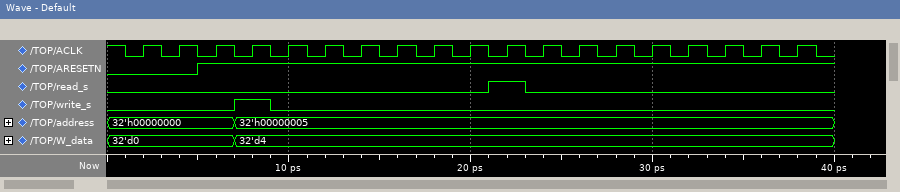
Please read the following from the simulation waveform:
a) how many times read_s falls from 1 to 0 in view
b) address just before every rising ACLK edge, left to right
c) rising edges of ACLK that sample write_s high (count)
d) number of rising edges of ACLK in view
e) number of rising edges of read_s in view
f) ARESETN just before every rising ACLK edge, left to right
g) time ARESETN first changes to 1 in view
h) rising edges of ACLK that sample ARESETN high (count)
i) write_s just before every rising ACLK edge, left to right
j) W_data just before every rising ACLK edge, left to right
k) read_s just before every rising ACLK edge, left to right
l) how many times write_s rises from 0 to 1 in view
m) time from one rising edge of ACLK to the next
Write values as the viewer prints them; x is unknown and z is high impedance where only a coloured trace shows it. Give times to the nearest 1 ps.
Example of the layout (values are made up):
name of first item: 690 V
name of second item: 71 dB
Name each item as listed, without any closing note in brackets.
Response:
how many times read_s falls from 1 to 0 in view: 1
address just before every rising ACLK edge, left to right: 32'h00000000, 32'h00000000, 32'h00000000, 32'h00000005, 32'h00000005, 32'h00000005, 32'h00000005, 32'h00000005, 32'h00000005, 32'h00000005, 32'h00000005, 32'h00000005, 32'h00000005, 32'h00000005, 32'h00000005, 32'h00000005, 32'h00000005, 32'h00000005, 32'h00000005
rising edges of ACLK that sample write_s high: 1
number of rising edges of ACLK in view: 19
number of rising edges of read_s in view: 1
ARESETN just before every rising ACLK edge, left to right: 0 0 1 1 1 1 1 1 1 1 1 1 1 1 1 1 1 1 1
time ARESETN first changes to 1 in view: 5 ps
rising edges of ACLK that sample ARESETN high: 17
write_s just before every rising ACLK edge, left to right: 0 0 0 1 0 0 0 0 0 0 0 0 0 0 0 0 0 0 0
W_data just before every rising ACLK edge, left to right: 32'd0, 32'd0, 32'd0, 32'd4, 32'd4, 32'd4, 32'd4, 32'd4, 32'd4, 32'd4, 32'd4, 32'd4, 32'd4, 32'd4, 32'd4, 32'd4, 32'd4, 32'd4, 32'd4
read_s just before every rising ACLK edge, left to right: 0 0 0 0 0 0 0 0 0 0 1 0 0 0 0 0 0 0 0
how many times write_s rises from 0 to 1 in view: 1
time from one rising edge of ACLK to the next: 2 ps
